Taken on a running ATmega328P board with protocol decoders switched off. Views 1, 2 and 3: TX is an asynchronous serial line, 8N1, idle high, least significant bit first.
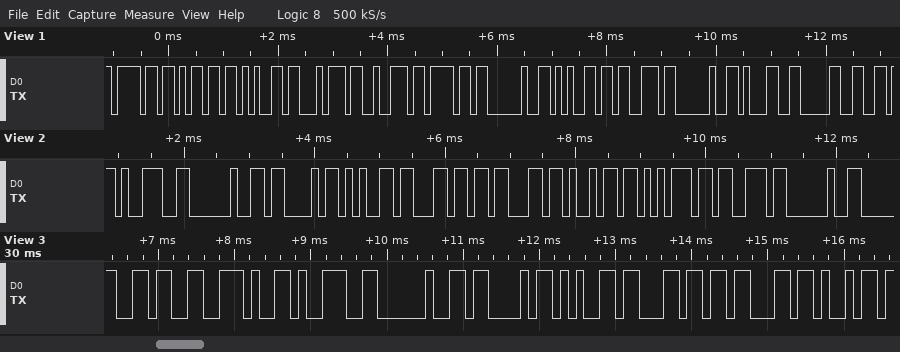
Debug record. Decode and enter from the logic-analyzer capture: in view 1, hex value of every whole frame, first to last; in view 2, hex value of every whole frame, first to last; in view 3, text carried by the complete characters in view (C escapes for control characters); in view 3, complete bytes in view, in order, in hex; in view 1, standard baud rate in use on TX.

6F 6D 65 74 72 6F 20 65 73 20 31 30
0x39 0x20 0x43 0x65 0x6C 0x63 0x69 0x75 0x73 0x20
"6.9 Celci"
0x36 0x2E 0x39 0x20 0x43 0x65 0x6C 0x63 0x69
9600 baud
